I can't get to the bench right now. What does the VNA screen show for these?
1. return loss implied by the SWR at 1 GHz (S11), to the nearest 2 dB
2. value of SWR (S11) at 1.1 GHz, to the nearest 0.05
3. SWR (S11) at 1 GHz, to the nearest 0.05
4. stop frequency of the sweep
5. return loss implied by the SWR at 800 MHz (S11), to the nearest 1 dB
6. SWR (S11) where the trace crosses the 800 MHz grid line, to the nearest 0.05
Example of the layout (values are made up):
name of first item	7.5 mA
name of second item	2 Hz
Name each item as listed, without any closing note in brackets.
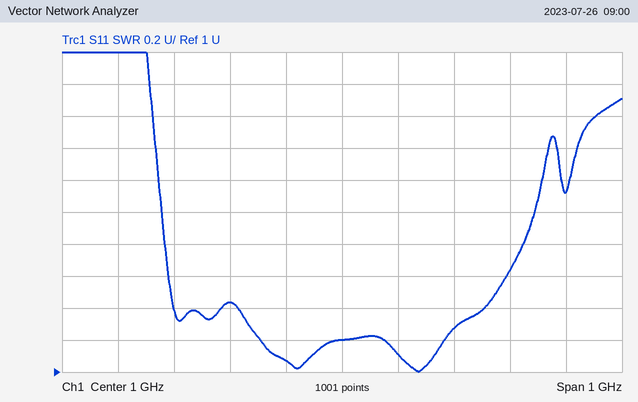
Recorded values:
return loss implied by the SWR at 1 GHz (S11), to the nearest 2 dB	20 dB
value of SWR (S11) at 1.1 GHz, to the nearest 0.05	1.10
SWR (S11) at 1 GHz, to the nearest 0.05	1.20
stop frequency of the sweep	1.5 GHz
return loss implied by the SWR at 800 MHz (S11), to the nearest 1 dB	15 dB
SWR (S11) where the trace crosses the 800 MHz grid line, to the nearest 0.05	1.45
